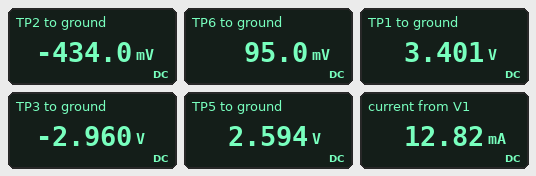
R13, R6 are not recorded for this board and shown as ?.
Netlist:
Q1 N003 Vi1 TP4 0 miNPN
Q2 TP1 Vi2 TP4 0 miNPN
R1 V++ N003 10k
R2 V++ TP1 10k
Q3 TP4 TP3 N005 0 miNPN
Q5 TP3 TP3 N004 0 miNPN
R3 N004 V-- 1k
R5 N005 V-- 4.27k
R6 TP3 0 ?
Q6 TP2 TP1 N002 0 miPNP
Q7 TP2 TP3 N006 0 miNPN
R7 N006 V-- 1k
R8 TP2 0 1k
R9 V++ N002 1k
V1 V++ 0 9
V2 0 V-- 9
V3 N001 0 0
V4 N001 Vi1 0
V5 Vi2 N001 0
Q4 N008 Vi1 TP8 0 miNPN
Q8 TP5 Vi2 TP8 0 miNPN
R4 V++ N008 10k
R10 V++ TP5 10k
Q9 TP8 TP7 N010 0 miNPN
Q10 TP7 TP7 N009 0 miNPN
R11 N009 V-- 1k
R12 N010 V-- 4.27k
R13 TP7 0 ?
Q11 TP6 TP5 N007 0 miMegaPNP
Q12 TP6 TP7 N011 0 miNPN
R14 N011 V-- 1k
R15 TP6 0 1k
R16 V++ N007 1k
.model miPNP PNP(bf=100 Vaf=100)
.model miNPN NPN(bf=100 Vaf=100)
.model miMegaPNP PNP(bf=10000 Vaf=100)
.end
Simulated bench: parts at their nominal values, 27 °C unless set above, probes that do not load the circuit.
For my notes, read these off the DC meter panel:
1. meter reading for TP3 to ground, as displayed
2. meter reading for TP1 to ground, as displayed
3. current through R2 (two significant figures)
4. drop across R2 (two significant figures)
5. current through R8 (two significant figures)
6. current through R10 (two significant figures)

-2.960 V
3.401 V
560 µA
5.6 V
430 µA
640 µA
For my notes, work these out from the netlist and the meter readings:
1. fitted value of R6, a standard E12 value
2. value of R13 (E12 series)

560 Ω
470 Ω
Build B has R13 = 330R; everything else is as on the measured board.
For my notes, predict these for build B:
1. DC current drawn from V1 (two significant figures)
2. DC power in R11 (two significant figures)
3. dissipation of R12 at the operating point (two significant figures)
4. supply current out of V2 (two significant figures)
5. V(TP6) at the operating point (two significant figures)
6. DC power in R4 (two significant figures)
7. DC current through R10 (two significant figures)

14 mA
38 mW
8.9 mW
25 mA
180 mV
5.0 mW
710 µA
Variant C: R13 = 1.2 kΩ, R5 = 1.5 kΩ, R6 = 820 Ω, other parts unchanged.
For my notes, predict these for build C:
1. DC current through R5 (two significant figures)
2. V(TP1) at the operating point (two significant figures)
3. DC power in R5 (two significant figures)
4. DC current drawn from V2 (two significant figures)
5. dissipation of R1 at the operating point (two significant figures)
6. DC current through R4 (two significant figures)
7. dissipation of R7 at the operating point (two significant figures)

3.0 mA
1.1 V
13 mW
20 mA
9.5 mW
430 µA
20 mW
